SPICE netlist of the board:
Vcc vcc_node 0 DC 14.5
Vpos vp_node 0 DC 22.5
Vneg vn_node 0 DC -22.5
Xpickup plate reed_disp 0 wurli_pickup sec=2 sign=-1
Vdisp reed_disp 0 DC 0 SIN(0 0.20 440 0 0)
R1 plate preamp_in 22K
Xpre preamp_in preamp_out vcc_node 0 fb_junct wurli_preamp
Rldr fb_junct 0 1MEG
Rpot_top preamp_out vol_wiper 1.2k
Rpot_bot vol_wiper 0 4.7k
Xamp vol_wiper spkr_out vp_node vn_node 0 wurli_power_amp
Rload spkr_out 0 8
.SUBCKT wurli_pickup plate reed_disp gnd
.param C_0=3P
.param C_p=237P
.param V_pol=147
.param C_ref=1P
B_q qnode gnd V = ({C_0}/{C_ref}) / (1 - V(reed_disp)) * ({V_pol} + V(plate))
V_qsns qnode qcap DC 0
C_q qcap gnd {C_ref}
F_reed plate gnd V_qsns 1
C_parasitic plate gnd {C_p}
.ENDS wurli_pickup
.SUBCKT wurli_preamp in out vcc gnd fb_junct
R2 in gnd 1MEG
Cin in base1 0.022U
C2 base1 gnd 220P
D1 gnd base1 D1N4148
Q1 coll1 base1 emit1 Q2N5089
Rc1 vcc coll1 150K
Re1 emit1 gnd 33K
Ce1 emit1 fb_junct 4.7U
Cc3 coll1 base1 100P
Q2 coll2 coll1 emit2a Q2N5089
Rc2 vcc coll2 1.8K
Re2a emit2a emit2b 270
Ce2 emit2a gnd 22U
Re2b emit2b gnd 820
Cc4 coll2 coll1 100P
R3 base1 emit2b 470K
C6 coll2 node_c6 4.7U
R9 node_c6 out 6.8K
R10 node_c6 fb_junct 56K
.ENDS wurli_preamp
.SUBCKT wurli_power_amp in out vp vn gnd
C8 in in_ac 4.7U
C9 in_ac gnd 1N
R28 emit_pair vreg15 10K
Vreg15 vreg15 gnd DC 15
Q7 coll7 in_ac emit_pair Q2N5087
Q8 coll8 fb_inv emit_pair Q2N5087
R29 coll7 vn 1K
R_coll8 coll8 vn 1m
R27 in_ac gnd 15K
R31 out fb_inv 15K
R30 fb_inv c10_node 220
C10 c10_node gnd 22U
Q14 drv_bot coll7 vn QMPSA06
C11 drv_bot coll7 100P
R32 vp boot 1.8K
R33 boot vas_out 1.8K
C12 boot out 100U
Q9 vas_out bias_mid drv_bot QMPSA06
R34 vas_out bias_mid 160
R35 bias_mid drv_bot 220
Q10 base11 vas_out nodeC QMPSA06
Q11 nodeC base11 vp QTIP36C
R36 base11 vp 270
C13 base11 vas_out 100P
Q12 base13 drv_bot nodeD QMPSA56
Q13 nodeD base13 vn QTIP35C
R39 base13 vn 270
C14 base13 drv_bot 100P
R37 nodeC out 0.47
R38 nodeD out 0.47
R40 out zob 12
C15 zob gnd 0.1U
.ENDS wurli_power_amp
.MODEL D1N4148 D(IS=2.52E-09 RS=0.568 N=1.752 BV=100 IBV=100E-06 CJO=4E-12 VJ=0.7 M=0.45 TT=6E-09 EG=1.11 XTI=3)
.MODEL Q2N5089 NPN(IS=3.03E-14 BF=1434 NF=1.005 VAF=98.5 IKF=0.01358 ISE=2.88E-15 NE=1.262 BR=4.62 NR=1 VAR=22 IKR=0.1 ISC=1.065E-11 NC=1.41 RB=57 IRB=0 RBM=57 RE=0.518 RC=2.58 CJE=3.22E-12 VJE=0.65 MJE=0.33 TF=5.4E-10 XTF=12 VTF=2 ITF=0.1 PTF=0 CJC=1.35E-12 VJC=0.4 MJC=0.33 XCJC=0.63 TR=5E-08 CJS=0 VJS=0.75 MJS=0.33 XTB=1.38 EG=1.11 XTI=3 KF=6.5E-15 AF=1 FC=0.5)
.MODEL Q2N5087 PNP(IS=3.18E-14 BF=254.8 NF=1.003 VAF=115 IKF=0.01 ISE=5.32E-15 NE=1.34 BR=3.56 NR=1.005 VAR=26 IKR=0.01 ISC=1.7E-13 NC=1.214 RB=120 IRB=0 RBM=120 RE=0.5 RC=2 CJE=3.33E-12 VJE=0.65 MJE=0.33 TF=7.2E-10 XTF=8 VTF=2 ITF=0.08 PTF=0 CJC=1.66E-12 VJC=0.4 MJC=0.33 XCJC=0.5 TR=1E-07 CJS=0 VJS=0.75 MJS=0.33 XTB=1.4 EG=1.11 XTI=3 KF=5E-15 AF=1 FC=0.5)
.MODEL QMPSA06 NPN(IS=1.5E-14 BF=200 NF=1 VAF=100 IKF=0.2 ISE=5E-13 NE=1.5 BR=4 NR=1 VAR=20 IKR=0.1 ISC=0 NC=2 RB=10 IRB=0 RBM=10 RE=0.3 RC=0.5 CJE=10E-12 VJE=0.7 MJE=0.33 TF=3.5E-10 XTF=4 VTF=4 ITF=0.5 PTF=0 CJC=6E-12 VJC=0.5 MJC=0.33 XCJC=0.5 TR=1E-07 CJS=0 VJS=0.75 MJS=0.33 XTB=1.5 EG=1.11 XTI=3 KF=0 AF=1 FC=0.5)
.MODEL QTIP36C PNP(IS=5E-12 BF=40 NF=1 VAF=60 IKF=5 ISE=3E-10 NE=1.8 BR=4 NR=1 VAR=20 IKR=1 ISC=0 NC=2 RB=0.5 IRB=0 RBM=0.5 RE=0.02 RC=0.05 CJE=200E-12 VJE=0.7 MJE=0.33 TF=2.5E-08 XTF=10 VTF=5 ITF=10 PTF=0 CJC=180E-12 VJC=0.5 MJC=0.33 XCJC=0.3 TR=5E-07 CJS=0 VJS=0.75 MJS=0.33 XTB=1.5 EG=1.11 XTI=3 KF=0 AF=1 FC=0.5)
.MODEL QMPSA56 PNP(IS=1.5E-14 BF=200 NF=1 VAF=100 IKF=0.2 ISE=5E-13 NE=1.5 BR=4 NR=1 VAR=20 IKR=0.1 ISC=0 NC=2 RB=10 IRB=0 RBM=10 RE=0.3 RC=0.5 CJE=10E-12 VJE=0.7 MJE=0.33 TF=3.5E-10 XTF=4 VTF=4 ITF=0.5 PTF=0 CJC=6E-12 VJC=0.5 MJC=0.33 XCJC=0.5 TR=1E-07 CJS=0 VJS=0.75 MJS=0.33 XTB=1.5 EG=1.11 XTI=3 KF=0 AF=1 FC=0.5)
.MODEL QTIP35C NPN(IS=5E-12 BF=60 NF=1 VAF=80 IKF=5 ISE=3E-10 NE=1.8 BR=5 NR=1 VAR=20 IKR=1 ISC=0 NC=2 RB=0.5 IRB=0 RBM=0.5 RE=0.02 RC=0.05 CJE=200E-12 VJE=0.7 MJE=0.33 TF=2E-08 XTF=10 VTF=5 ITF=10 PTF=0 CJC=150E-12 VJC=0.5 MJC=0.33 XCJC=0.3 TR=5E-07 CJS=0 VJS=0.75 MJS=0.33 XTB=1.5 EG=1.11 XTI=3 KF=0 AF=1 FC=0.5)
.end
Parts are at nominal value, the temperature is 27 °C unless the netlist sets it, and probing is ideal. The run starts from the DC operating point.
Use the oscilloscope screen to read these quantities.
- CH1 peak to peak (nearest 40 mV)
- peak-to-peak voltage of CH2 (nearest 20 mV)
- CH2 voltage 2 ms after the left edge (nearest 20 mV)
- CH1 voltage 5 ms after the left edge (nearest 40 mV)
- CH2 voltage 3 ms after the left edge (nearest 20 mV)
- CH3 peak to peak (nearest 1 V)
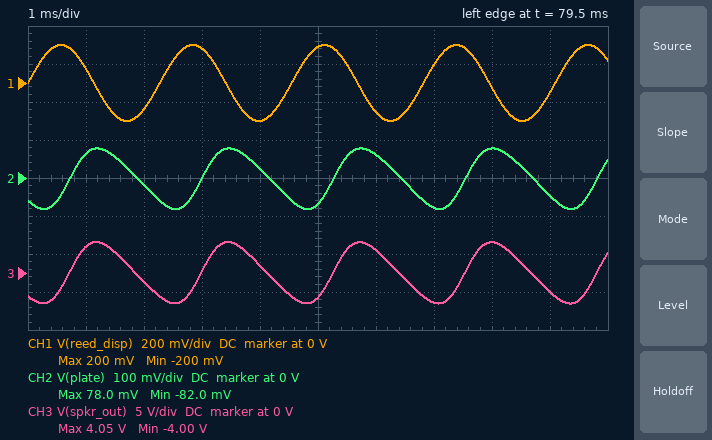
400 mV
160 mV
-20 mV
200 mV
0 V
8 V
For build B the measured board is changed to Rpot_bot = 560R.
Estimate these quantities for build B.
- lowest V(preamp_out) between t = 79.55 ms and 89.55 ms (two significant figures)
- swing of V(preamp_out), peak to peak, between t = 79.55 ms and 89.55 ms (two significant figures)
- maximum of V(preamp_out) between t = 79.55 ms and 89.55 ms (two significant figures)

-39 mV
77 mV
38 mV
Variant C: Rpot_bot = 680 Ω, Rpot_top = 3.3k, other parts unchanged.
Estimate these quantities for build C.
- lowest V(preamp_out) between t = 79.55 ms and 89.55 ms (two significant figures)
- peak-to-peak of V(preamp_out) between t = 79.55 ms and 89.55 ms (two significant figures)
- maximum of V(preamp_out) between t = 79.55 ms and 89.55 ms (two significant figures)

-71 mV
140 mV
69 mV
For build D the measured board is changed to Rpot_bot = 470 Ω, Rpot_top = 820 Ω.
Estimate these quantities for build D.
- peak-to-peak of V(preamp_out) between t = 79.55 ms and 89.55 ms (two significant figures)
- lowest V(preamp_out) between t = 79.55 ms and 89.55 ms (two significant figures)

60 mV
-30 mV
